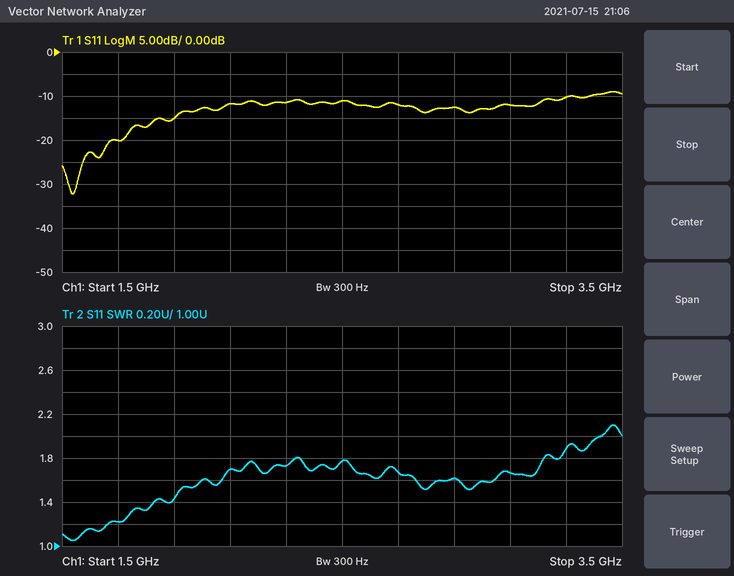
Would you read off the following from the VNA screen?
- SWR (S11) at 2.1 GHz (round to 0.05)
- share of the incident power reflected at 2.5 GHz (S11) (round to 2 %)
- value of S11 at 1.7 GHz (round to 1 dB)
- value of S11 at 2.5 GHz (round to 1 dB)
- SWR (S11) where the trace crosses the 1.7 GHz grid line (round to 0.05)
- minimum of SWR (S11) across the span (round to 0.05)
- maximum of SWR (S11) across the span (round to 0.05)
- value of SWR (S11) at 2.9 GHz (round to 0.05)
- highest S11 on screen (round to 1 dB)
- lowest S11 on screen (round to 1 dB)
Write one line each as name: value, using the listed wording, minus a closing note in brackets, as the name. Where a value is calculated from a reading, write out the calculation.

SWR (S11) at 2.1 GHz: 1.70
share of the incident power reflected at 2.5 GHz (S11): 10^(-11/10) ≈ 8 %
value of S11 at 1.7 GHz: -20 dB
value of S11 at 2.5 GHz: -11 dB
SWR (S11) where the trace crosses the 1.7 GHz grid line: 1.20
minimum of SWR (S11) across the span: 1.05
maximum of SWR (S11) across the span: 2.10
value of SWR (S11) at 2.9 GHz: 1.60
highest S11 on screen: -9 dB
lowest S11 on screen: -32 dB
